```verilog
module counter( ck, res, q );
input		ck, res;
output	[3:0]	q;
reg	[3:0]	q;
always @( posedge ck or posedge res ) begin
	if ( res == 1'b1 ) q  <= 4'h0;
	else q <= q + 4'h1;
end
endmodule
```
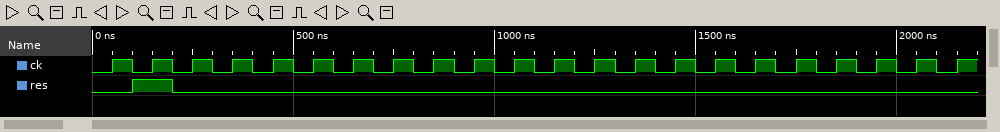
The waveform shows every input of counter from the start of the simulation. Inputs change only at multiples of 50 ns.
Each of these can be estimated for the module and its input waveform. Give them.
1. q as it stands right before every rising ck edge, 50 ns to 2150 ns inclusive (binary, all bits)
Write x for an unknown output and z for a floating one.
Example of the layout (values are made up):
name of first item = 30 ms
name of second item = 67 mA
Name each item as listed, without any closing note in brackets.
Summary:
q as it stands right before every rising ck edge, 50 ns to 2150 ns inclusive = x, 0000, 0000, 0001, 0010, 0011, 0100, 0101, 0110, 0111, 1000, 1001, 1010, 1011, 1100, 1101, 1110, 1111, 0000, 0001, 0010, 0011
